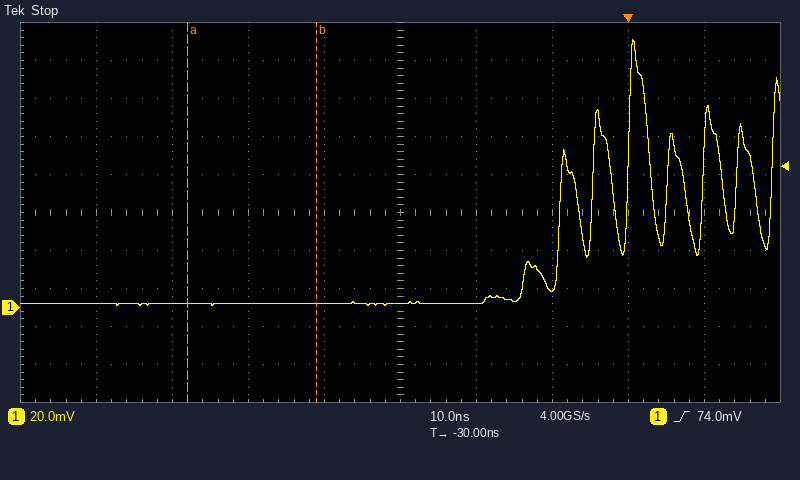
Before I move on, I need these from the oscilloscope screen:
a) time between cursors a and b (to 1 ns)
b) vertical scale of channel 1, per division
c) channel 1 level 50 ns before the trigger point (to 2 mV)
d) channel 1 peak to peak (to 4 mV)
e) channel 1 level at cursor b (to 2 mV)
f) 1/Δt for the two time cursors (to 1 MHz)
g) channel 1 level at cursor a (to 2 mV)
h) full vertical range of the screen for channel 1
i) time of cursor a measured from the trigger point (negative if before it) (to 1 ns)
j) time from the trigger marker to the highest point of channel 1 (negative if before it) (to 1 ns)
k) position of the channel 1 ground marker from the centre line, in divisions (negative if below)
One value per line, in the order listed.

17 ns
20 mV
2 mV
140 mV
2 mV
59 MHz
2 mV
200 mV
-58 ns
+1 ns
-2.5 div
